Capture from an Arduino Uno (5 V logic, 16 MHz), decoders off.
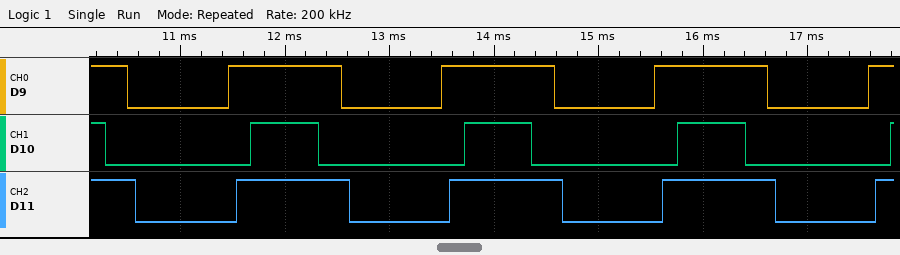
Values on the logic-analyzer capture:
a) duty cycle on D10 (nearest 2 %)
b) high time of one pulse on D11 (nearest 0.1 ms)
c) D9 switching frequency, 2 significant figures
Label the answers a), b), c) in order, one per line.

a) 32 %
b) 1.1 ms
c) 490 Hz
